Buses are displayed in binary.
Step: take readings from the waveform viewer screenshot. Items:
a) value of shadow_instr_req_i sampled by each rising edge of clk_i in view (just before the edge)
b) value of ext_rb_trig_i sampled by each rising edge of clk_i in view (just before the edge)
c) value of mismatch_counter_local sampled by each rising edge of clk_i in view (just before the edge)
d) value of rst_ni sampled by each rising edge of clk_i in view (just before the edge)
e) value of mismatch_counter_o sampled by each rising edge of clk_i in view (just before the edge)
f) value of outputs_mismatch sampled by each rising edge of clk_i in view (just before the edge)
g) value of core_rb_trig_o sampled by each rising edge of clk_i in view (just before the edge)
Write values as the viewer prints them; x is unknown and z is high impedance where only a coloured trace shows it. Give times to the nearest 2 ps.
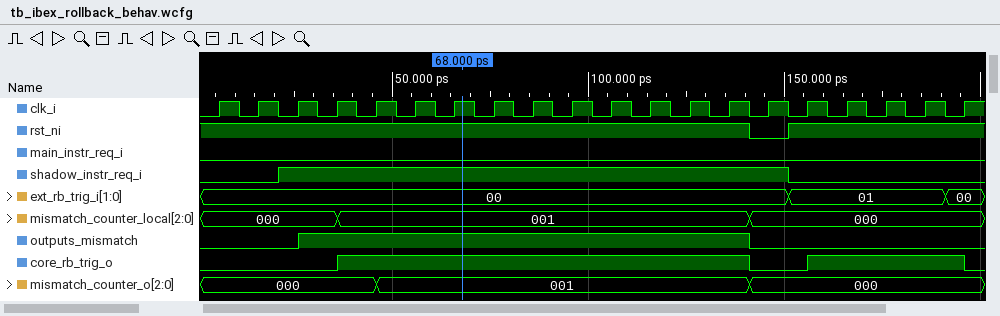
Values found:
0 0 1 1 1 1 1 1 1 1 1 1 1 1 1 0 0 0 0 0
00, 00, 00, 00, 00, 00, 00, 00, 00, 00, 00, 00, 00, 00, 00, 01, 01, 01, 01, 00
000, 000, 000, 000, 001, 001, 001, 001, 001, 001, 001, 001, 001, 001, 000, 000, 000, 000, 000, 000
1 1 1 1 1 1 1 1 1 1 1 1 1 1 0 1 1 1 1 1
000, 000, 000, 000, 000, 001, 001, 001, 001, 001, 001, 001, 001, 001, 000, 000, 000, 000, 000, 000
0 0 0 1 1 1 1 1 1 1 1 1 1 1 0 0 0 0 0 0
0 0 0 0 1 1 1 1 1 1 1 1 1 1 0 0 1 1 1 1
